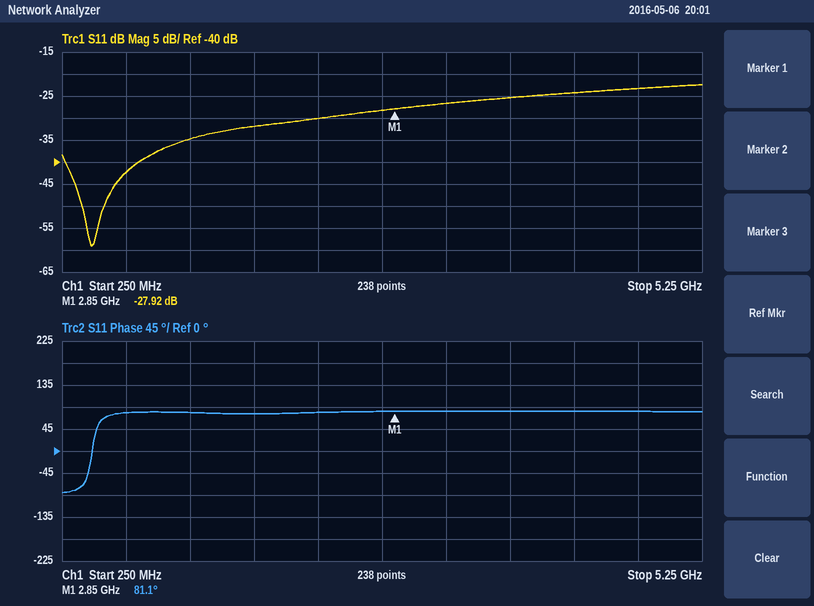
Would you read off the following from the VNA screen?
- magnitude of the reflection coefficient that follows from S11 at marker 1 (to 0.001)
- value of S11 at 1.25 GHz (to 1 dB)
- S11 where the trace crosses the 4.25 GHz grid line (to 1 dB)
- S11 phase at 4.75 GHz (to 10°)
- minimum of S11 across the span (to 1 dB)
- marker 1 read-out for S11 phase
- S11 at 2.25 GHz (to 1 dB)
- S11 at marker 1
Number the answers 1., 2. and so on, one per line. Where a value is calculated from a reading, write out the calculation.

1. 10^(-27.92/20) ≈ 0.040
2. -35 dB
3. -24 dB
4. 80°
5. -59 dB
6. 81.1°
7. -30 dB
8. -27.92 dB
